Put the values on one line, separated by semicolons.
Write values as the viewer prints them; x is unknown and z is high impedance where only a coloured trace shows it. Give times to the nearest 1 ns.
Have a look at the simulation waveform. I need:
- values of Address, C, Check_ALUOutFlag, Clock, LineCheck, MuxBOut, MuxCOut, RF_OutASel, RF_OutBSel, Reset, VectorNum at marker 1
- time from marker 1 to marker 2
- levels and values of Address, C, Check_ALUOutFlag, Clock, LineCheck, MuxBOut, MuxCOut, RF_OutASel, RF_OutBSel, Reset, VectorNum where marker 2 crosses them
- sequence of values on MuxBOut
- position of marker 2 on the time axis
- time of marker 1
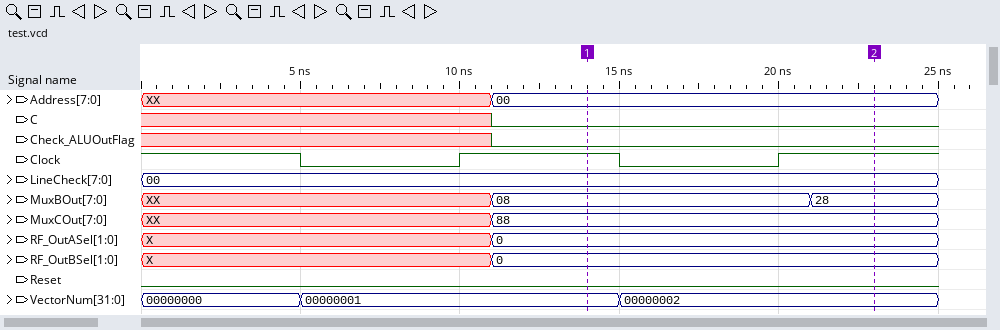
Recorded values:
Address=00, C=0, Check_ALUOutFlag=0, Clock=1, LineCheck=00, MuxBOut=08, MuxCOut=88, RF_OutASel=0, RF_OutBSel=0, Reset=0, VectorNum=00000001; 9 ns; Address=00, C=0, Check_ALUOutFlag=0, Clock=1, LineCheck=00, MuxBOut=28, MuxCOut=88, RF_OutASel=0, RF_OutBSel=0, Reset=0, VectorNum=00000002; XX, 08, 28; 23 ns; 14 ns
